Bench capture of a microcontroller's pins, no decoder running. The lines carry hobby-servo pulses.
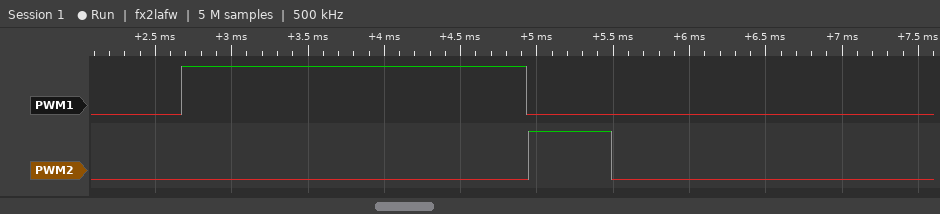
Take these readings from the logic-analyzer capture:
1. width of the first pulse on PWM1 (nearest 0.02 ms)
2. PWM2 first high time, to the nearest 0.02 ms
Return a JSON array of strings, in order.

["2.26 ms", "0.54 ms"]
